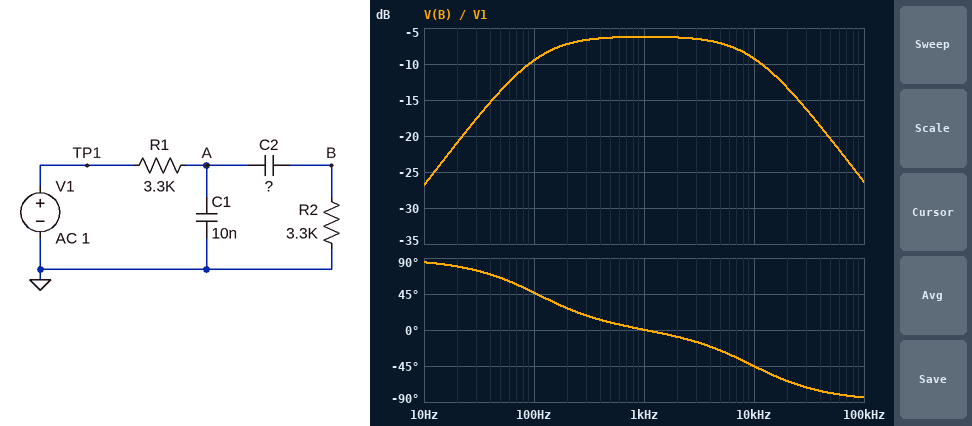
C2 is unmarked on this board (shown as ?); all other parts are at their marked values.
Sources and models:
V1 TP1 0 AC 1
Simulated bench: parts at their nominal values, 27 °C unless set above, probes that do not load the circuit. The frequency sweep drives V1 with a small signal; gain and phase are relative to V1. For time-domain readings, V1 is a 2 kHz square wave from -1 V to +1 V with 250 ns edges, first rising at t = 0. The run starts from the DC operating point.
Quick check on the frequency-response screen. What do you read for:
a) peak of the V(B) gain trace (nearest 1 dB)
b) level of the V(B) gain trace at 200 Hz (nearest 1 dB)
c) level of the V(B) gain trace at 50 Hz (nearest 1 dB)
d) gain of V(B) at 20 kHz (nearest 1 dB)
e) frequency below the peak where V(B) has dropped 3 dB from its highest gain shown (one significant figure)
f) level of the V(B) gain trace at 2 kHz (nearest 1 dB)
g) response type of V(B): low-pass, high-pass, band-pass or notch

-6 dB
-7 dB
-14 dB
-13 dB
100 Hz
-6 dB
band-pass
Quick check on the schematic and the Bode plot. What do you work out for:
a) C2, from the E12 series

220 nF
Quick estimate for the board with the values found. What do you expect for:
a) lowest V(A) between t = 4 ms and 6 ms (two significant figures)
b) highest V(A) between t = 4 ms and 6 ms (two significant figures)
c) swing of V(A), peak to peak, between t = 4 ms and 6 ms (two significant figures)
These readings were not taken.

-560 mV
520 mV
1.1 V
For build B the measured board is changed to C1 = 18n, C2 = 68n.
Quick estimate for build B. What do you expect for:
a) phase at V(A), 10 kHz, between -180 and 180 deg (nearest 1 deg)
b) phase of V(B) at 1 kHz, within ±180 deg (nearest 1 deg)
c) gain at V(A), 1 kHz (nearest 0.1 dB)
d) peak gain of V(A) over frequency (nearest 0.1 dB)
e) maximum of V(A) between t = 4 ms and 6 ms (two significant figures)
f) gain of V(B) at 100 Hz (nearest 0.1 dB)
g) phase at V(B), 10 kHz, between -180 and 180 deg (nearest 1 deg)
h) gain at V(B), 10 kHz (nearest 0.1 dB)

-62 deg
8 deg
-5.4 dB
0 dB
580 mV
-17.4 dB
-58 deg
-12.7 dB
